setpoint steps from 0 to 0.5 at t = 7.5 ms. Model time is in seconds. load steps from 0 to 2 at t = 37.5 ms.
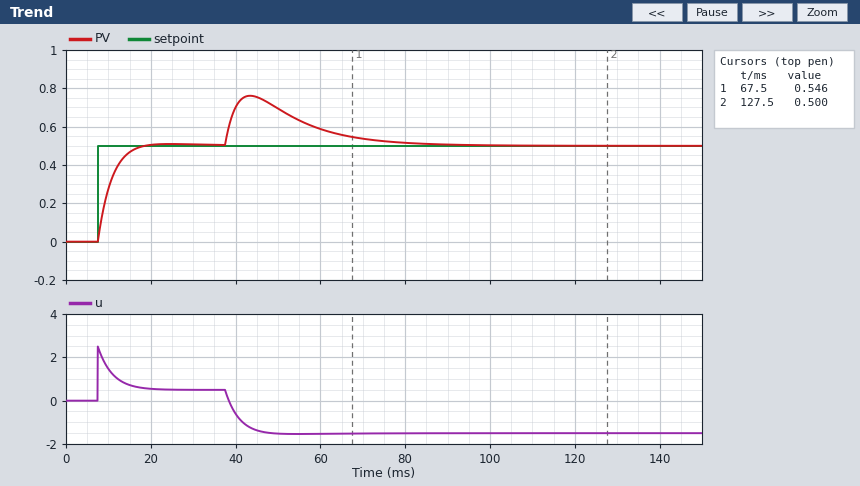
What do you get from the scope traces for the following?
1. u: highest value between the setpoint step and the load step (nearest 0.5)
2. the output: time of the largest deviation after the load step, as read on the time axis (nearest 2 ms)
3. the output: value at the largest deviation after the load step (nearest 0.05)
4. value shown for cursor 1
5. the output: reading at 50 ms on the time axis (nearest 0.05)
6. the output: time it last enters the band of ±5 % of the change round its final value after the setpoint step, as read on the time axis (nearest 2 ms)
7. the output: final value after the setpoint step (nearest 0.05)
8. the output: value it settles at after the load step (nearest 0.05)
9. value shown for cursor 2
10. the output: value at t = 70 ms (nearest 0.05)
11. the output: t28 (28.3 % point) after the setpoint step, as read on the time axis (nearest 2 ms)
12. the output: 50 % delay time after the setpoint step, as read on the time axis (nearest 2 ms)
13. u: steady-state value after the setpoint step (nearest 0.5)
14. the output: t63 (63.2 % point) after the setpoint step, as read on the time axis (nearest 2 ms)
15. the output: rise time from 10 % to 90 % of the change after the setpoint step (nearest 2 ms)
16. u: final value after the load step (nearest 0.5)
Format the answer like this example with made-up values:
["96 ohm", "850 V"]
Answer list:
["2.5", "44 ms", "0.75", "0.546", "0.70", "16 ms", "0.50", "0.50", "0.500", "0.55", "8 ms", "10 ms", "0.5", "10 ms", "6 ms", "-1.5"]
